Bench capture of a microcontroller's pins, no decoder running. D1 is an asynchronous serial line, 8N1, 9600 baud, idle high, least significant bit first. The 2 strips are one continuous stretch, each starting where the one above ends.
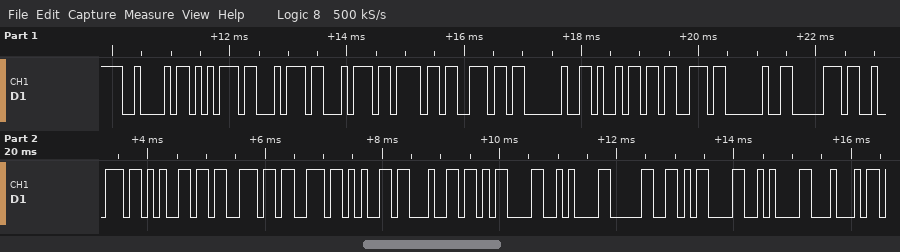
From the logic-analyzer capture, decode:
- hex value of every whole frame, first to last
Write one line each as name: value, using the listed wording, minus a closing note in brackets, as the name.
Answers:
hex value of every whole frame, first to last: 0x42 0x75 0x74 0x74 0x6F 0x6E 0x20 0x69 0x73 0x20 0x70 0x72 0x65 0x73 0x73 0x65 0x64 0x0D 0x0A 0x30 0x0D 0x0A 0x44
